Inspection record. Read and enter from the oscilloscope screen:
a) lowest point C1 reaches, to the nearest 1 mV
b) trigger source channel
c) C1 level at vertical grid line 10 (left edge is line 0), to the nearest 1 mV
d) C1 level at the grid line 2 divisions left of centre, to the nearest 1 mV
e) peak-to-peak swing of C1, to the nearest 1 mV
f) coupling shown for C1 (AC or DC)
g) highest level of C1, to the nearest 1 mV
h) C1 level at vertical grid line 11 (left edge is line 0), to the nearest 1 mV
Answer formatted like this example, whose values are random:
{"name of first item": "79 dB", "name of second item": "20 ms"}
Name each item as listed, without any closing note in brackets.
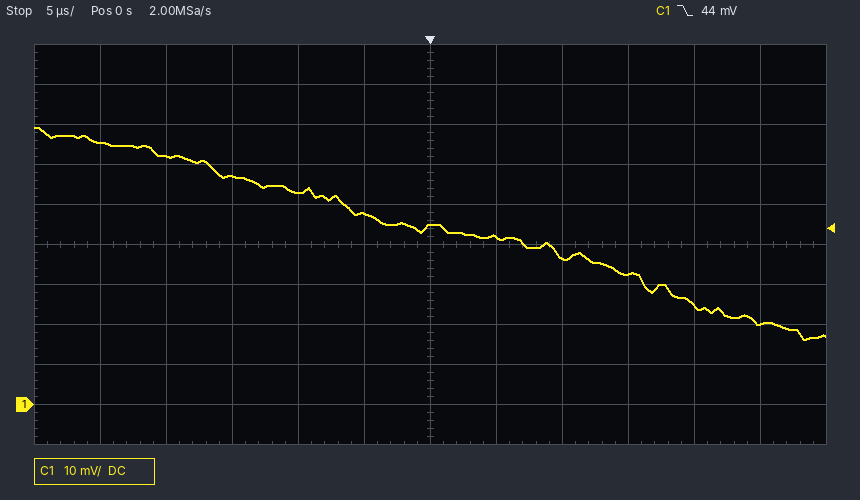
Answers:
{"lowest point C1 reaches, to the nearest 1 mV": "16 mV", "trigger source channel": "C1", "C1 level at vertical grid line 10 (left edge is line 0), to the nearest 1 mV": "25 mV", "C1 level at the grid line 2 divisions left of centre, to the nearest 1 mV": "53 mV", "peak-to-peak swing of C1, to the nearest 1 mV": "53 mV", "coupling shown for C1": "DC", "highest level of C1, to the nearest 1 mV": "69 mV", "C1 level at vertical grid line 11 (left edge is line 0), to the nearest 1 mV": "20 mV"}
